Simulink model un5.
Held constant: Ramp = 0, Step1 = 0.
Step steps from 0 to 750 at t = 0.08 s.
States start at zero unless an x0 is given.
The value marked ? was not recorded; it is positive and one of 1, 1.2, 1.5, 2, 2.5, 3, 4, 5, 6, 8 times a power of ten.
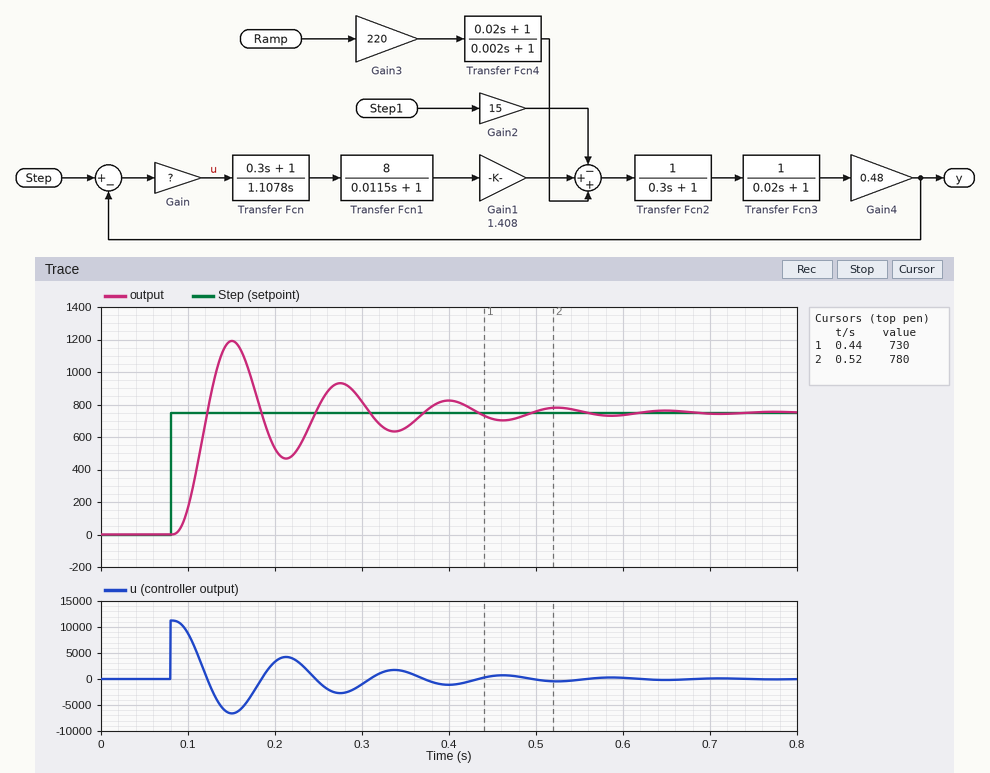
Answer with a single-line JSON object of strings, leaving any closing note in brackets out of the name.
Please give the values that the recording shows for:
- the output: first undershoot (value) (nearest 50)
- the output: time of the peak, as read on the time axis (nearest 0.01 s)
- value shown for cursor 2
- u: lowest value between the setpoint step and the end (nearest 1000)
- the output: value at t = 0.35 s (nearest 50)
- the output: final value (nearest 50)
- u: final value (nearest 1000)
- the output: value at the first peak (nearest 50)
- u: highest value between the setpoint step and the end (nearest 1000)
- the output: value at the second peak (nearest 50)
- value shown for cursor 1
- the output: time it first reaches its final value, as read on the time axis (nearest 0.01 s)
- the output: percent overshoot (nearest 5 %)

{"the output: first undershoot (value)": "450", "the output: time of the peak, as read on the time axis": "0.15 s", "value shown for cursor 2": "780", "u: lowest value between the setpoint step and the end": "-7000", "the output: value at t = 0.35 s": "650", "the output: final value": "750", "u: final value": "0", "the output: value at the first peak": "1200", "u: highest value between the setpoint step and the end": "11000", "the output: value at the second peak": "950", "value shown for cursor 1": "730", "the output: time it first reaches its final value, as read on the time axis": "0.12 s", "the output: percent overshoot": "60 %"}
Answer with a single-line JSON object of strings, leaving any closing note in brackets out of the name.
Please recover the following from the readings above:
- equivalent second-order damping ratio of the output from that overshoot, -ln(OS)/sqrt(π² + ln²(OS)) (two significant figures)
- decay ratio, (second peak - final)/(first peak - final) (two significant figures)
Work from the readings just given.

{"equivalent second-order damping ratio of the output from that overshoot, -ln(OS)/sqrt(π² + ln²(OS))": "0.16", "decay ratio, (second peak - final)/(first peak - final)": "0.44"}
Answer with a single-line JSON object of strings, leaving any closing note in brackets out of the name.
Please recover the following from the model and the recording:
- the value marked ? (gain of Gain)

{"the value marked ?": "15"}
